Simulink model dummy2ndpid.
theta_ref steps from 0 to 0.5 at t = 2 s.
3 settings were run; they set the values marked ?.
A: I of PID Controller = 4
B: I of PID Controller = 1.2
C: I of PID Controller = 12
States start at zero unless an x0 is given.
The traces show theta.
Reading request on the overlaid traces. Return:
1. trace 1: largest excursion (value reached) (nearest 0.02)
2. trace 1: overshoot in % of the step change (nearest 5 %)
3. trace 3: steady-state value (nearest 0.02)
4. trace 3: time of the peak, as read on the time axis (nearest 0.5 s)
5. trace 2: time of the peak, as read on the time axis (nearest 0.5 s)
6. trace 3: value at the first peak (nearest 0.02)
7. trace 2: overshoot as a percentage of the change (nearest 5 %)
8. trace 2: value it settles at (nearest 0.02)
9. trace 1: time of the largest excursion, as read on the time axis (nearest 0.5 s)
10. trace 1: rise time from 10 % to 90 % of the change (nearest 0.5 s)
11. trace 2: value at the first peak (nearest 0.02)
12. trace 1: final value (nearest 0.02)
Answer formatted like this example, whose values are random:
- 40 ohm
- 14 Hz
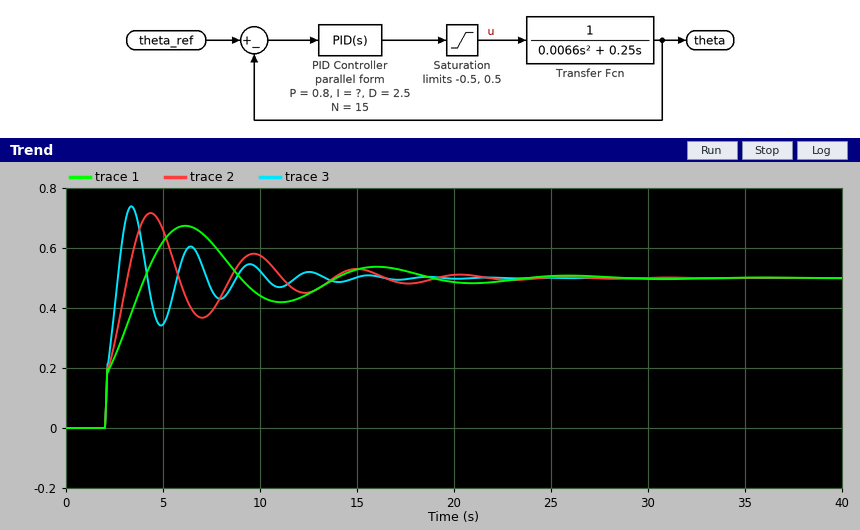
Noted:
- 0.68
- 35 %
- 0.50
- 3.5 s
- 4.5 s
- 0.74
- 45 %
- 0.50
- 6.0 s
- 1.5 s
- 0.72
- 0.50
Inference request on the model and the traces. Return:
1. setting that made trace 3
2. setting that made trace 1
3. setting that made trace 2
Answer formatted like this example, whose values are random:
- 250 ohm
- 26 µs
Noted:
- C
- B
- A
